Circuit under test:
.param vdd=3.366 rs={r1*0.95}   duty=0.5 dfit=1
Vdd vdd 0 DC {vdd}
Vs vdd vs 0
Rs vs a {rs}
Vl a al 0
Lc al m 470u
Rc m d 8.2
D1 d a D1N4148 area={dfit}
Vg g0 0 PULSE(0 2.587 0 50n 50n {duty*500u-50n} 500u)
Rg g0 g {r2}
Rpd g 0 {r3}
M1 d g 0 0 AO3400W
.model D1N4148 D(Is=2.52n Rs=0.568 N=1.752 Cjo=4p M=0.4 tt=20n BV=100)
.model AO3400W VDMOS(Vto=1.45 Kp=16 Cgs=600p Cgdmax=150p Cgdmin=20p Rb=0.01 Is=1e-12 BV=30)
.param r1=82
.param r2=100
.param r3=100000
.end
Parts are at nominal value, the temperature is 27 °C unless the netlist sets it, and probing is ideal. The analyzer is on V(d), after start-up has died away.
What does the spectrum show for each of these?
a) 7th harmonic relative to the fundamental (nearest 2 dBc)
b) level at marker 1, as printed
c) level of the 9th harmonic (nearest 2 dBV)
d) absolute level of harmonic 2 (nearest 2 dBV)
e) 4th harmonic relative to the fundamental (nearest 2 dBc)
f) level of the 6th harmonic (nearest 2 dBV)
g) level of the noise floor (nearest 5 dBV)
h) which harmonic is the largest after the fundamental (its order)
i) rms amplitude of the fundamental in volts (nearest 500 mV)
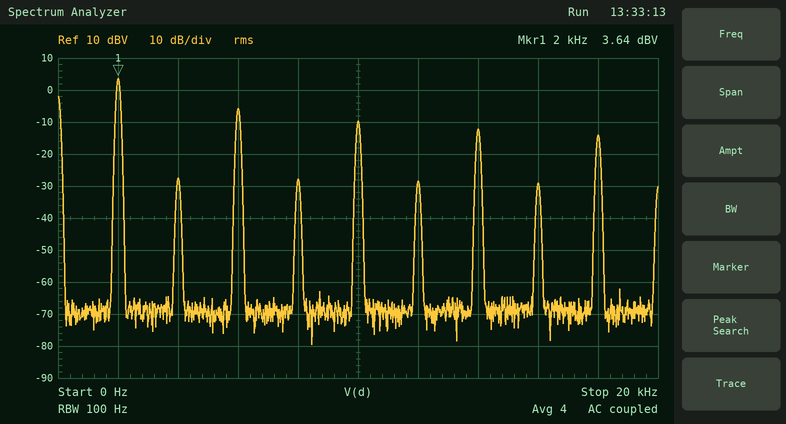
-16 dBc
3.64 dBV
-14 dBV
-28 dBV
-32 dBc
-28 dBV
-70 dBV
3
1.5 V
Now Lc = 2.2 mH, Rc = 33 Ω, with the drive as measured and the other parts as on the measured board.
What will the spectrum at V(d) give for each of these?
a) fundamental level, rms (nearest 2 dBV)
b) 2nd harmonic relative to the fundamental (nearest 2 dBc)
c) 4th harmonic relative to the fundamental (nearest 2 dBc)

4 dBV
-24 dBc
-26 dBc
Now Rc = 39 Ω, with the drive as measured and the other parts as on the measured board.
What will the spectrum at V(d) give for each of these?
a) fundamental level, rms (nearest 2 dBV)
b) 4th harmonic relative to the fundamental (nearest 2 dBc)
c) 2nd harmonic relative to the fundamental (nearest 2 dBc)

4 dBV
-36 dBc
-36 dBc
